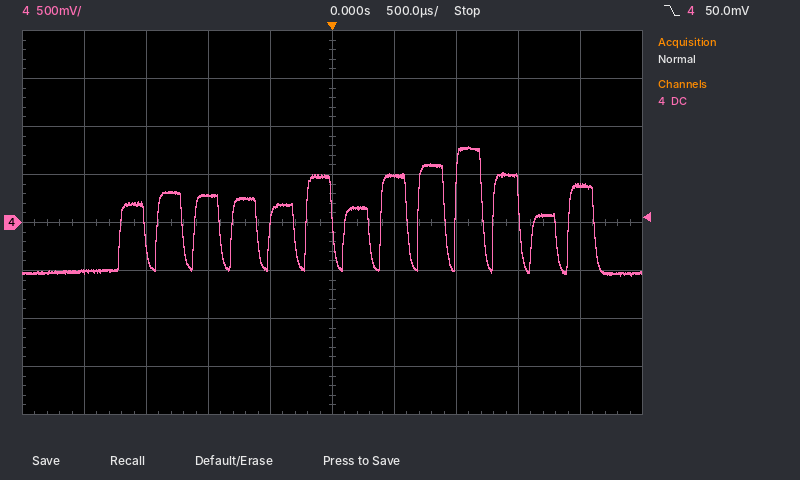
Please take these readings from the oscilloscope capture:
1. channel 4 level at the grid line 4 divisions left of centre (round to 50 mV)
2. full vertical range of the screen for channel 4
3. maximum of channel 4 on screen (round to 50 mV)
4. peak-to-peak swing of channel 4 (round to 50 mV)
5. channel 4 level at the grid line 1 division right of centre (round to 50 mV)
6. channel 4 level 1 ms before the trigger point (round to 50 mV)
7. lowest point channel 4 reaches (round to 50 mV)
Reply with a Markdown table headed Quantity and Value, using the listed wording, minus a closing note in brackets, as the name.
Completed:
| Quantity | Value |
|---|---|
| channel 4 level at the grid line 4 divisions left of centre | -500 mV |
| full vertical range of the screen for channel 4 | 4 V |
| maximum of channel 4 on screen | 800 mV |
| peak-to-peak swing of channel 4 | 1.35 V |
| channel 4 level at the grid line 1 division right of centre | 500 mV |
| channel 4 level 1 ms before the trigger point | 300 mV |
| lowest point channel 4 reaches | -550 mV |
